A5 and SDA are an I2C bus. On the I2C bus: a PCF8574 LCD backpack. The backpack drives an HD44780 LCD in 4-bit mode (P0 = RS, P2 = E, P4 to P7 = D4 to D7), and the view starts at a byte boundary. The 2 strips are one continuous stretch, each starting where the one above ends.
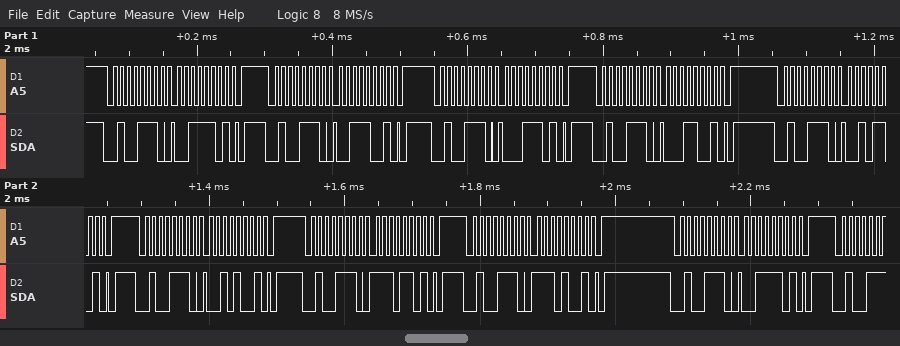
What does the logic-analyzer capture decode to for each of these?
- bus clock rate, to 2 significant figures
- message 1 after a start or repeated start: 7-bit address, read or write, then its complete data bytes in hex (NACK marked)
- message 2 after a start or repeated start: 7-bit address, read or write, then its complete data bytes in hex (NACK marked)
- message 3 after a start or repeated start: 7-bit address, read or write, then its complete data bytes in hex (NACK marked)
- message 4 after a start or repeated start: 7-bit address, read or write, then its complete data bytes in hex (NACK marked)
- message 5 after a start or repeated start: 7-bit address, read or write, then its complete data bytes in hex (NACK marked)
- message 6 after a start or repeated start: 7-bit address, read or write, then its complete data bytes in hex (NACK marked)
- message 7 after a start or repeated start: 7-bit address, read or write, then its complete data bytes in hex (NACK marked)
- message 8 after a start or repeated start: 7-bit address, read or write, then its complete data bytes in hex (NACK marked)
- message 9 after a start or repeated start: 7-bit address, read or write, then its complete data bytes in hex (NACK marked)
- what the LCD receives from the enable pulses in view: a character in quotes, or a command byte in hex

100 kHz
0x27 write: 3D
0x27 write: 39
0x27 write: 1D
0x27 write: 19
0x27 write: 2D
0x27 write: 29
0x27 write: ED
0x27 write: E9
0x27 write: 3D
'1' '.'
